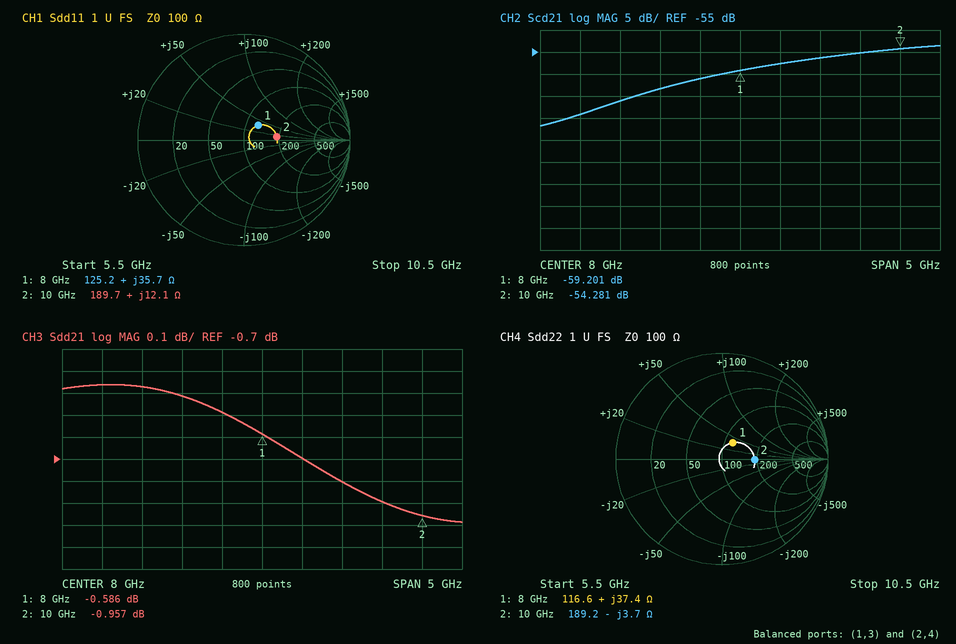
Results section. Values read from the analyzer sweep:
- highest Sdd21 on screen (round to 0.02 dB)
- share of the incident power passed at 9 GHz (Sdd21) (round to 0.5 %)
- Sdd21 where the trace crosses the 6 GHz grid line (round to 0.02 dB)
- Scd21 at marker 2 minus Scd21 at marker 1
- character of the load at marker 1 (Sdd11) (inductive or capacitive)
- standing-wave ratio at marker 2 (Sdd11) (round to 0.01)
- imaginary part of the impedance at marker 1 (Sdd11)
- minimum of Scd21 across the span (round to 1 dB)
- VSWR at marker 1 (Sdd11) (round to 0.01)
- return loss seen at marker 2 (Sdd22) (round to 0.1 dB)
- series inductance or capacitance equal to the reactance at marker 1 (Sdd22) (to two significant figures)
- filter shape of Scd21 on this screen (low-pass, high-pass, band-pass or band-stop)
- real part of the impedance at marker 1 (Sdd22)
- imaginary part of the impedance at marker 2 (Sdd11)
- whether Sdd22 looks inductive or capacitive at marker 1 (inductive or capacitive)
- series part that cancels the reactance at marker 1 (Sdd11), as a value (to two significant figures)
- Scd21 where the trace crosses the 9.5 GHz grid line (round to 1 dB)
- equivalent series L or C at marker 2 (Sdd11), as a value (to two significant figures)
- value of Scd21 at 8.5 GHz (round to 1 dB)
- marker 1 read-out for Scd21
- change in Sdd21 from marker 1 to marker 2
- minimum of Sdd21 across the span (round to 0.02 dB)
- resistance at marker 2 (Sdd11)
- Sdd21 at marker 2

-0.36 dB
83.0 %
-0.36 dB
4.920 dB
inductive
1.91
+35.7 Ω
-72 dB
1.47
10.2 dB
740 pH
high-pass
116.6 Ω
+12.1 Ω
inductive
560 fF
-55 dB
190 pH
-58 dB
-59.201 dB
-0.371 dB
-0.98 dB
189.7 Ω
-0.957 dB
